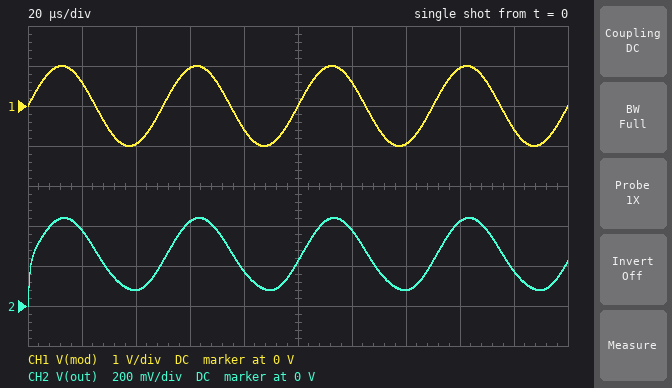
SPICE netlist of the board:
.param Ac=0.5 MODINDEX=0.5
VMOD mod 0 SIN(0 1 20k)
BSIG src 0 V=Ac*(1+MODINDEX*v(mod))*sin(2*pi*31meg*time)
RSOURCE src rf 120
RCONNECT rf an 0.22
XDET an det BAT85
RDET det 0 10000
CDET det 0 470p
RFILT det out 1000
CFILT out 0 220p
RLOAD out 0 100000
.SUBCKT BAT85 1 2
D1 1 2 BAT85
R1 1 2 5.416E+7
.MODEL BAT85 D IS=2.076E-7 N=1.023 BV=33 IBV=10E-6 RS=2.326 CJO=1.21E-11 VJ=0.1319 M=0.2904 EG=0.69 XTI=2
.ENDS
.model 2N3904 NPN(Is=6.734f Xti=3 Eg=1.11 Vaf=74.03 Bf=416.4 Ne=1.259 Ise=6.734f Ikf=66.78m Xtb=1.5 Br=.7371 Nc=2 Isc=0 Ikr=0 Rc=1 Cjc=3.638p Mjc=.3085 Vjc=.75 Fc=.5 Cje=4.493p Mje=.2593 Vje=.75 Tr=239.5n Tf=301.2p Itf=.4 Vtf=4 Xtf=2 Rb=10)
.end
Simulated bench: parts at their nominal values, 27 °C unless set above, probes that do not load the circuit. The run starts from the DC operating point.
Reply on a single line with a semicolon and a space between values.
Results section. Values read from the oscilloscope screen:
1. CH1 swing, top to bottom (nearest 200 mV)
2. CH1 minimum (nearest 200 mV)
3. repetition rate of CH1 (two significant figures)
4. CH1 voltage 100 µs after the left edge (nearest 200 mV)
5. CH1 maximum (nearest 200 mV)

2.0 V; -1.0 V; 20 kHz; 0 V; 1.0 V
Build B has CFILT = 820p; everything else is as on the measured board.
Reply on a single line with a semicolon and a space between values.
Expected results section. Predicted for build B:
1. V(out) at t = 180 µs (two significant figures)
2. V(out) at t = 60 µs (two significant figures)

220 mV; 410 mV
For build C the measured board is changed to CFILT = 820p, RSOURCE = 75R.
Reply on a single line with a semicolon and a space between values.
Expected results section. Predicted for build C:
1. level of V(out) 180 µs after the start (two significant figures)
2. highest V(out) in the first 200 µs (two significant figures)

230 mV; 460 mV
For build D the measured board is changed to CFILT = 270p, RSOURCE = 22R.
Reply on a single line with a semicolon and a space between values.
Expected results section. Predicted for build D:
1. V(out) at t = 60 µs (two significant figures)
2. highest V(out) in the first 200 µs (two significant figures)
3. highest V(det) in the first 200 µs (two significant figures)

480 mV; 500 mV; 520 mV
